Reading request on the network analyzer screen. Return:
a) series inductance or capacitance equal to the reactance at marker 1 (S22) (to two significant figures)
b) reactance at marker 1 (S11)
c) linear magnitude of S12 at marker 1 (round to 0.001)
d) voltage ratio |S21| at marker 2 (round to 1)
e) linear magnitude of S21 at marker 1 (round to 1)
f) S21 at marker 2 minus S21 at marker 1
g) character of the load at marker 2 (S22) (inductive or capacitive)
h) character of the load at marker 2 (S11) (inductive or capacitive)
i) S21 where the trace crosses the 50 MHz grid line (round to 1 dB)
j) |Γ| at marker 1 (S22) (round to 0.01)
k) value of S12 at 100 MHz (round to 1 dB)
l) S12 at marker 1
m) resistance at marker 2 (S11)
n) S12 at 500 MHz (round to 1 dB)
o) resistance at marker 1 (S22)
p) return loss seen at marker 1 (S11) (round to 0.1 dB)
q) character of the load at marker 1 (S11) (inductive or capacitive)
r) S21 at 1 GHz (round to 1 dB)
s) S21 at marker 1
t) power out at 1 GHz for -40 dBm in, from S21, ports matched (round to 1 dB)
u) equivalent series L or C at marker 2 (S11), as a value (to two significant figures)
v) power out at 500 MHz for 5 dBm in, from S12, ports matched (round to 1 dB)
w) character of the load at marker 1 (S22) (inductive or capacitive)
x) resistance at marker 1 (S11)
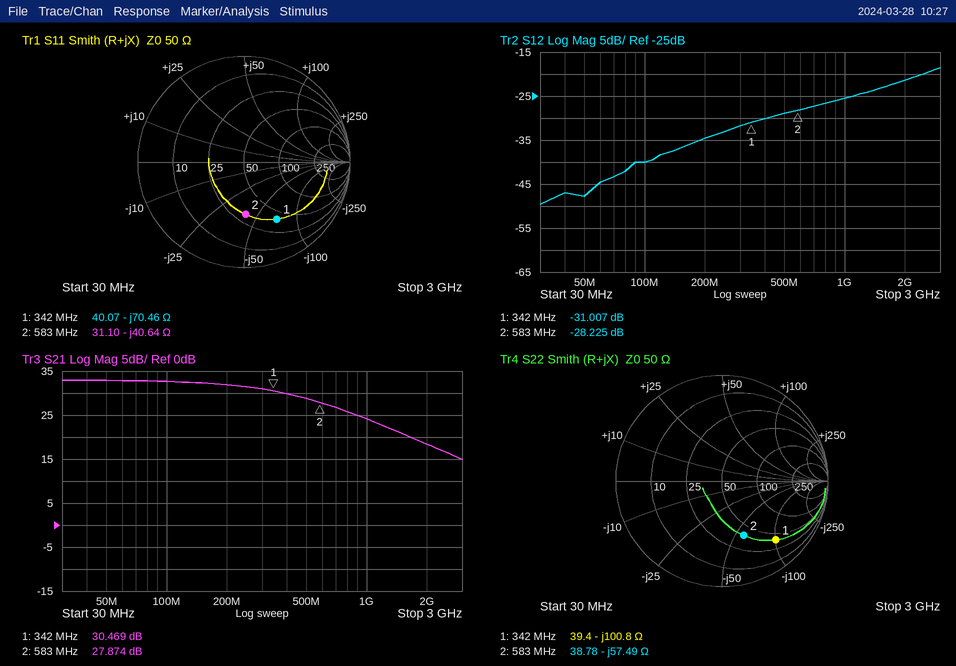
4.6 pF
-70.46 Ω
0.028
25
33
-2.595 dB
capacitive
capacitive
33 dB
0.75
-40 dB
-31.007 dB
31.10 Ω
-29 dB
39.4 Ω
4.1 dB
capacitive
24 dB
30.469 dB
-16 dBm
6.7 pF
-24 dBm
capacitive
40.07 Ω
